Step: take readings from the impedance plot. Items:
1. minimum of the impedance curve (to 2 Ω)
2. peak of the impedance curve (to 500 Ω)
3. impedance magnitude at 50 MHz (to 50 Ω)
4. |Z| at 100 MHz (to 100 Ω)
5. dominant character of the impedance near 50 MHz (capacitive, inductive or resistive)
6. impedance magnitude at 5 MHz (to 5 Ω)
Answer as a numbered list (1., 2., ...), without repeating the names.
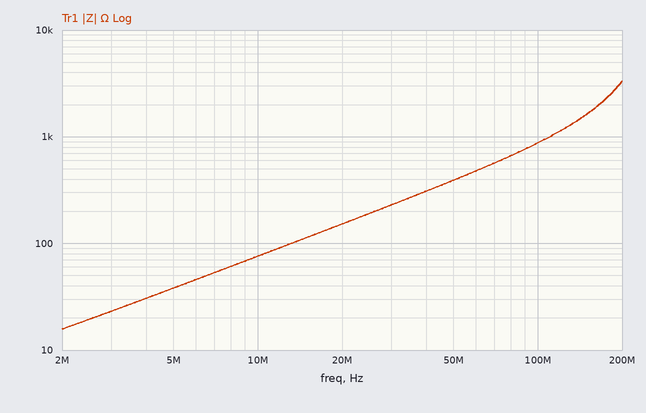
1. 16 Ω
2. 3.5 kΩ
3. 400 Ω
4. 900 Ω
5. inductive
6. 40 Ω
